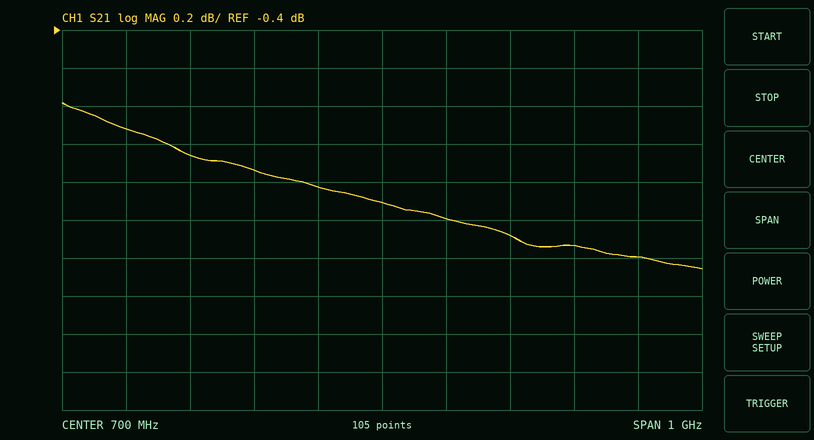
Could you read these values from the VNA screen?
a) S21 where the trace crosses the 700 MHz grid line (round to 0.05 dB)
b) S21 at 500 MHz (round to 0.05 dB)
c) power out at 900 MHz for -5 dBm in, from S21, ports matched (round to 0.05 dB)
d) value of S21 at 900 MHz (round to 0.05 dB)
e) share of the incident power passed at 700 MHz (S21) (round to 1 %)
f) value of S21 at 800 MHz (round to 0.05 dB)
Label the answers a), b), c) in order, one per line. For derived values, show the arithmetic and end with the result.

a) -1.30 dB
b) -1.15 dB
c) -5 dBm + (-1.50 dB) = -6.50 dBm
d) -1.50 dB
e) 10^(-1.3/10) ≈ 74 %
f) -1.40 dB
